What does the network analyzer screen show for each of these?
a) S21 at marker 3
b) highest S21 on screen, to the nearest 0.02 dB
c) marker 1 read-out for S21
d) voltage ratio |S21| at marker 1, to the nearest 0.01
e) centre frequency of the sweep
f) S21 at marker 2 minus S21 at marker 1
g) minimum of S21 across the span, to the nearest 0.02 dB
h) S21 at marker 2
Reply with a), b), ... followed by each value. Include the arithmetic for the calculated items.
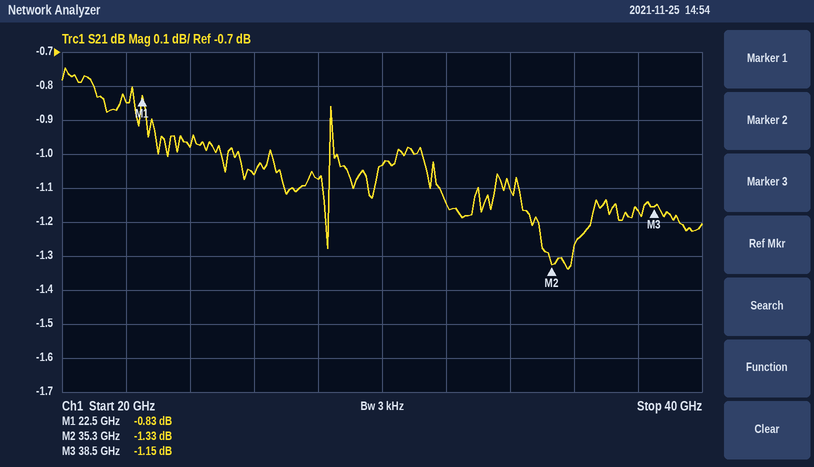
a) -1.15 dB
b) -0.74 dB
c) -0.83 dB
d) 10^(-0.83/20) ≈ 0.91
e) 30 GHz
f) -1.33 − (-0.83) = -0.50 dB
g) -1.34 dB
h) -1.33 dB
